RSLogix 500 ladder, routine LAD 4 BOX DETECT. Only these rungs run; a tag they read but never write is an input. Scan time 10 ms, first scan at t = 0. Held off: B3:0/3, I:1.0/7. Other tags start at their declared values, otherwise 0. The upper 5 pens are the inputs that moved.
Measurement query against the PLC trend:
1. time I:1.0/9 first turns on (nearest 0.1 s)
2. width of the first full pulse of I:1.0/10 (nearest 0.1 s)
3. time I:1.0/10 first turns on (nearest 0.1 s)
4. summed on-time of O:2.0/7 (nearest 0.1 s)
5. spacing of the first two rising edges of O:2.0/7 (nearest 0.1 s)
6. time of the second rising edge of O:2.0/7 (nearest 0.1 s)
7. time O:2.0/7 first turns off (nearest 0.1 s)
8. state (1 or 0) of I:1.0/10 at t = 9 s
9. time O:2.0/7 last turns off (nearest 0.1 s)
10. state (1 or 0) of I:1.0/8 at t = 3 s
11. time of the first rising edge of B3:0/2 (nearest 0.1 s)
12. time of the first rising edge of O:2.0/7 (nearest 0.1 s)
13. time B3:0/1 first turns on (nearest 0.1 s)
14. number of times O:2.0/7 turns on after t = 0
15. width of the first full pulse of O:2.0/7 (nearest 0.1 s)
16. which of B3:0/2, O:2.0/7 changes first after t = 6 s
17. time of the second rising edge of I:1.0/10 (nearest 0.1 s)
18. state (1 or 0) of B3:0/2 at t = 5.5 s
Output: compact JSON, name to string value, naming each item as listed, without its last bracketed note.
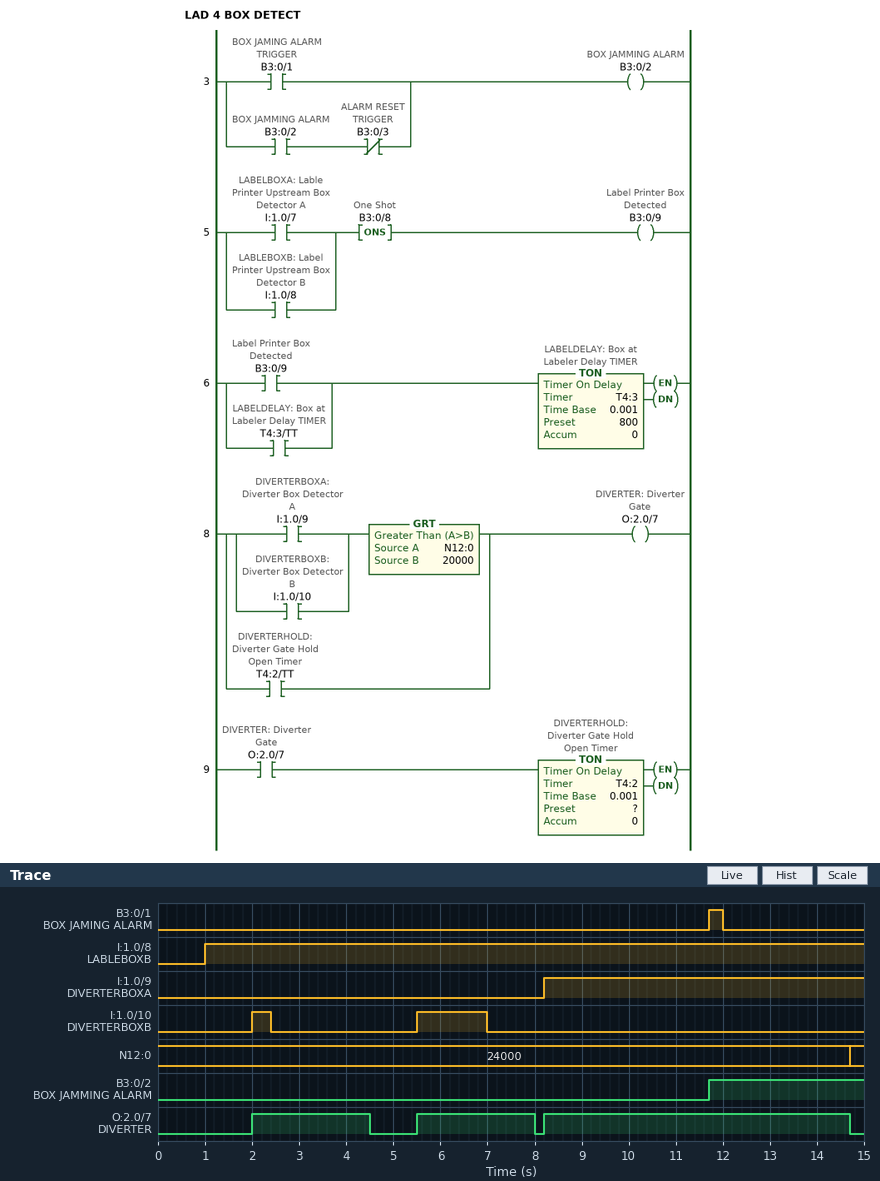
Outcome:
{"time I:1.0/9 first turns on": "8.2 s", "width of the first full pulse of I:1.0/10": "0.4 s", "time I:1.0/10 first turns on": "2.0 s", "summed on-time of O:2.0/7": "11.5 s", "spacing of the first two rising edges of O:2.0/7": "3.5 s", "time of the second rising edge of O:2.0/7": "5.5 s", "time O:2.0/7 first turns off": "4.5 s", "state (1 or 0) of I:1.0/10 at t = 9 s": "0", "time O:2.0/7 last turns off": "14.7 s", "state (1 or 0) of I:1.0/8 at t = 3 s": "1", "time of the first rising edge of B3:0/2": "11.7 s", "time of the first rising edge of O:2.0/7": "2.0 s", "time B3:0/1 first turns on": "11.7 s", "number of times O:2.0/7 turns on after t = 0": "3", "width of the first full pulse of O:2.0/7": "2.5 s", "which of B3:0/2, O:2.0/7 changes first after t = 6 s": "O:2.0/7", "time of the second rising edge of I:1.0/10": "5.5 s", "state (1 or 0) of B3:0/2 at t = 5.5 s": "0"}
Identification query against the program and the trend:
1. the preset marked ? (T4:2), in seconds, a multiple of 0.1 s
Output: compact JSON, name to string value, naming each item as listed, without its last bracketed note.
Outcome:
{"the preset marked ? (T4:2), in seconds, a multiple of 0.1 s": "2.5 s"}
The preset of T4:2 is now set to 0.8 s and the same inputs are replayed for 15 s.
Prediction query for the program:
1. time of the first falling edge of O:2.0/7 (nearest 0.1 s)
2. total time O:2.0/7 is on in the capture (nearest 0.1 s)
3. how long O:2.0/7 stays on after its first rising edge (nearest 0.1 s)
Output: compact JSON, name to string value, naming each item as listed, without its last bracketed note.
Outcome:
{"time of the first falling edge of O:2.0/7": "2.8 s", "total time O:2.0/7 is on in the capture": "8.8 s", "how long O:2.0/7 stays on after its first rising edge": "0.8 s"}
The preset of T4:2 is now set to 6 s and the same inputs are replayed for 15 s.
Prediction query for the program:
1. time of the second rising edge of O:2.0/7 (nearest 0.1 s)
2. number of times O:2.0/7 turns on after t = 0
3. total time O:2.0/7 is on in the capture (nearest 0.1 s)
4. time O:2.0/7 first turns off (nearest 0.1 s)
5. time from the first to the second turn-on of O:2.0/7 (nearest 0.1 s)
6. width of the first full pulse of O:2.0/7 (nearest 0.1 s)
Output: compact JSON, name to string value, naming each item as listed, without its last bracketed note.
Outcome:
{"time of the second rising edge of O:2.0/7": "8.2 s", "number of times O:2.0/7 turns on after t = 0": "2", "total time O:2.0/7 is on in the capture": "12.5 s", "time O:2.0/7 first turns off": "8.0 s", "time from the first to the second turn-on of O:2.0/7": "6.2 s", "width of the first full pulse of O:2.0/7": "6.0 s"}
